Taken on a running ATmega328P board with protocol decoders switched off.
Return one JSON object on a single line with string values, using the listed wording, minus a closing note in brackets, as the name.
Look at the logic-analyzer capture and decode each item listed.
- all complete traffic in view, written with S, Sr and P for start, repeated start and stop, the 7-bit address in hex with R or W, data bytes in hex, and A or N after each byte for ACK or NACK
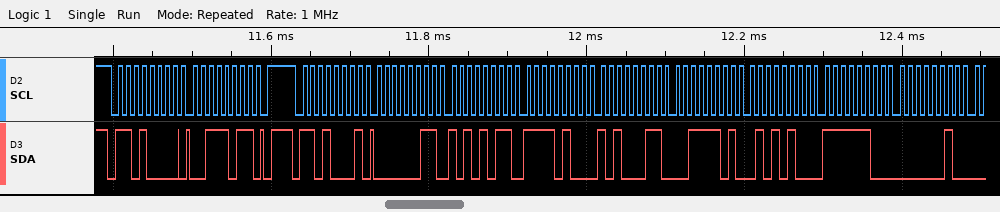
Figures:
{"all complete traffic in view, written with S, Sr and P for start, repeated start and stop, the 7-bit address in hex with R or W, data bytes in hex, and A or N after each byte for ACK or NACK": "S 68W A 3B A P S 68R A 03 A AB A F4 A A3 A 3D A 54 A FC A 02 A"}
